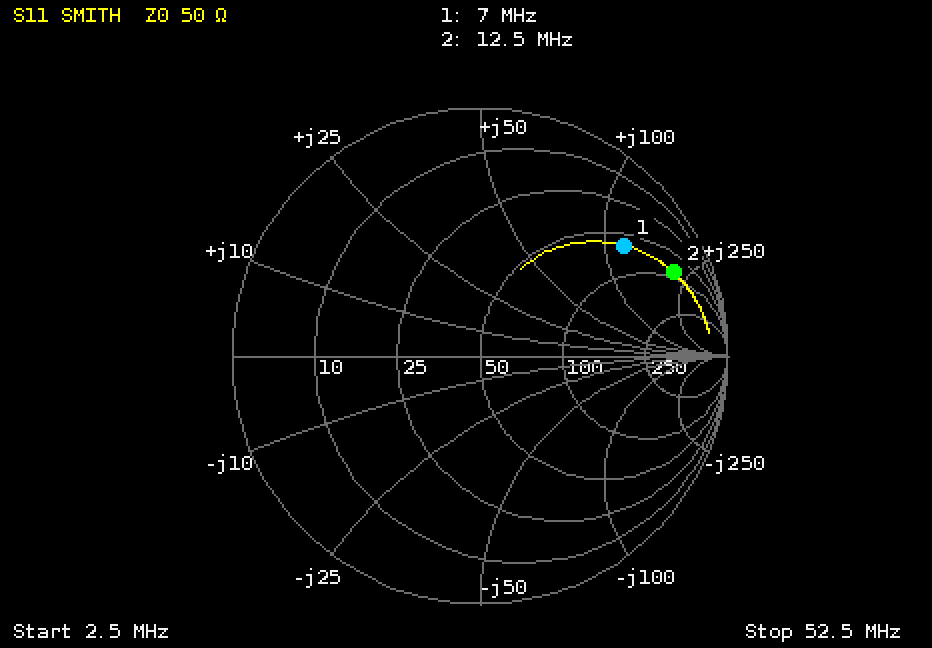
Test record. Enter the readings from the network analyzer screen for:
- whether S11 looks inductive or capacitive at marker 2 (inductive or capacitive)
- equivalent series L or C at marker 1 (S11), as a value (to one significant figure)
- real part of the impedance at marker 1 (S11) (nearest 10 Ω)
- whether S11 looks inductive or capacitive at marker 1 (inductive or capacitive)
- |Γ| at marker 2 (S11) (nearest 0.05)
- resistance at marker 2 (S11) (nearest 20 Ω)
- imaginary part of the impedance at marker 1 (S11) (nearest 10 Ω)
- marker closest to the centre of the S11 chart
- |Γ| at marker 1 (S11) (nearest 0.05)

inductive
3 µH
60 Ω
inductive
0.85
80 Ω
+120 Ω
marker 1
0.75
